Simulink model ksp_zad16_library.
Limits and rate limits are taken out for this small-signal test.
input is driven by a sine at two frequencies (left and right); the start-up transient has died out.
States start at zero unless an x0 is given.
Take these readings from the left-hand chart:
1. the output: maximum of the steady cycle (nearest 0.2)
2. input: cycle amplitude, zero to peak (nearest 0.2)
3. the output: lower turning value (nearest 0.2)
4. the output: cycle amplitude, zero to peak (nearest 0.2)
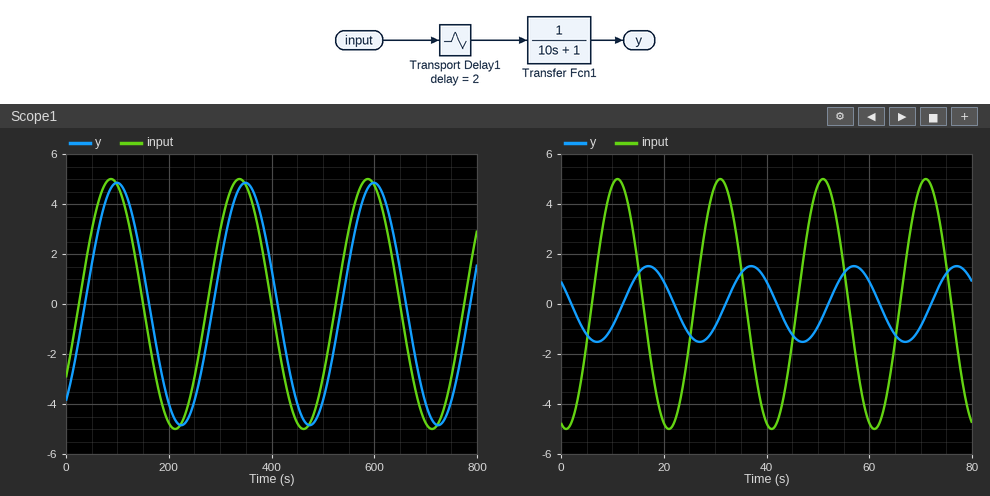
4.8
5.0
-4.8
4.8
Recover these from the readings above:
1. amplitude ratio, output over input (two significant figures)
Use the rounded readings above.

0.96
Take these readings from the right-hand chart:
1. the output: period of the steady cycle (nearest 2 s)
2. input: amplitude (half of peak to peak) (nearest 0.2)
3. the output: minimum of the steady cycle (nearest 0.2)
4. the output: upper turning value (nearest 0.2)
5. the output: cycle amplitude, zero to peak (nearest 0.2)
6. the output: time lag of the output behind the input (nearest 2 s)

20 s
5.0
-1.6
1.6
1.6
6 s
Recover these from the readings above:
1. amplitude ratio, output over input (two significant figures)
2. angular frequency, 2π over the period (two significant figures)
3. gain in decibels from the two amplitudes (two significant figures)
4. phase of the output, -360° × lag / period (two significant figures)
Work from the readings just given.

0.32
0.31 rad/s
-9.9 dB
-110°
